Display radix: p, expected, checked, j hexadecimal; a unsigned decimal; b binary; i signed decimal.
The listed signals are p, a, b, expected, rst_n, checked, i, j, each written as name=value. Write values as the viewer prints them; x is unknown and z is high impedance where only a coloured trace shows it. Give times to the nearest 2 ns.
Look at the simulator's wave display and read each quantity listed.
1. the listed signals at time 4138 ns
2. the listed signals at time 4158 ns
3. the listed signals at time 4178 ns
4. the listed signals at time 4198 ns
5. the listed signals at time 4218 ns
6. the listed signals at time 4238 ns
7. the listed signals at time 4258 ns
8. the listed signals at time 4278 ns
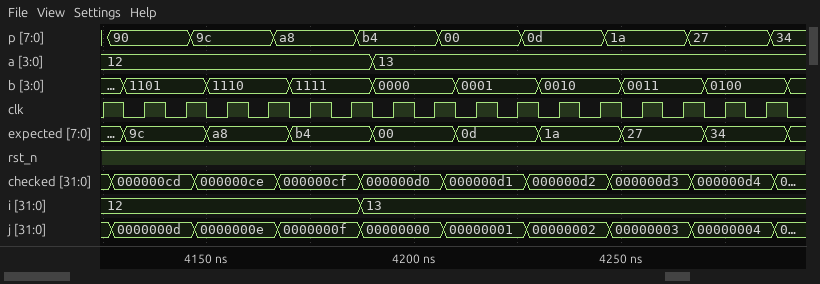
p=90, a=12, b=1101, expected=9c, rst_n=1, checked=000000cd, i=12, j=0000000d
p=9c, a=12, b=1110, expected=a8, rst_n=1, checked=000000ce, i=12, j=0000000e
p=a8, a=12, b=1111, expected=b4, rst_n=1, checked=000000cf, i=12, j=0000000f
p=b4, a=13, b=0000, expected=00, rst_n=1, checked=000000d0, i=13, j=00000000
p=00, a=13, b=0001, expected=0d, rst_n=1, checked=000000d1, i=13, j=00000001
p=0d, a=13, b=0010, expected=1a, rst_n=1, checked=000000d2, i=13, j=00000002
p=1a, a=13, b=0011, expected=27, rst_n=1, checked=000000d3, i=13, j=00000003
p=27, a=13, b=0100, expected=34, rst_n=1, checked=000000d4, i=13, j=00000004
